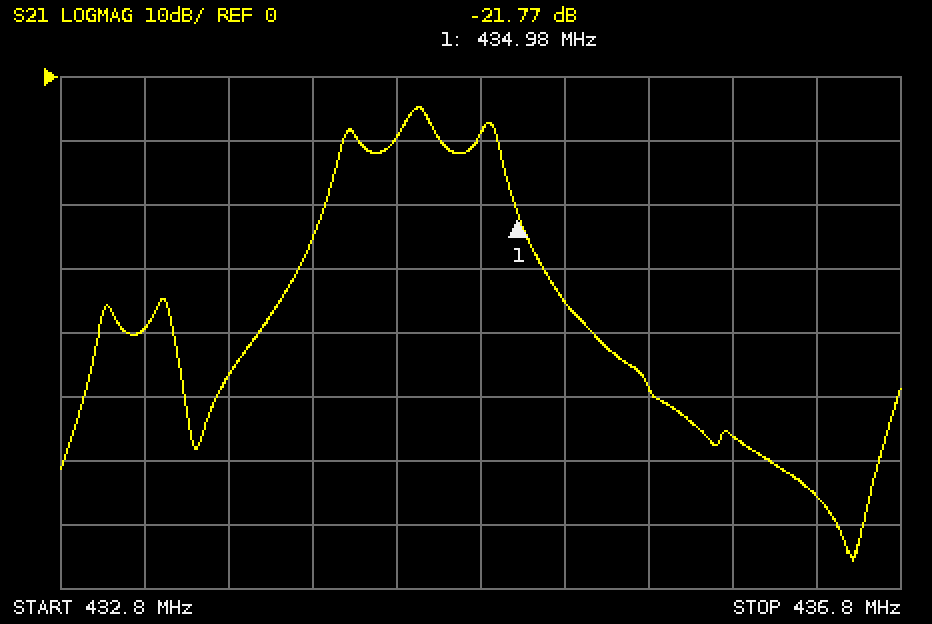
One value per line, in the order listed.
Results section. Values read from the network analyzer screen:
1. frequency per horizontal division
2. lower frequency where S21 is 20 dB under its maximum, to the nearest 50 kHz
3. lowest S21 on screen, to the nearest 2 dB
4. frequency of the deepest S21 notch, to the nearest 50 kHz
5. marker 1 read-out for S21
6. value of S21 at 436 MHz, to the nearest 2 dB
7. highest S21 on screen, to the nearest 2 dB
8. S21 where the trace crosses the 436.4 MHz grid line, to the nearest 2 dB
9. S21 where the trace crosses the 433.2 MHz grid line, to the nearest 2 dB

400 kHz
434.00 MHz
-76 dB
436.55 MHz
-21.77 dB
-56 dB
-4 dB
-66 dB
-40 dB
